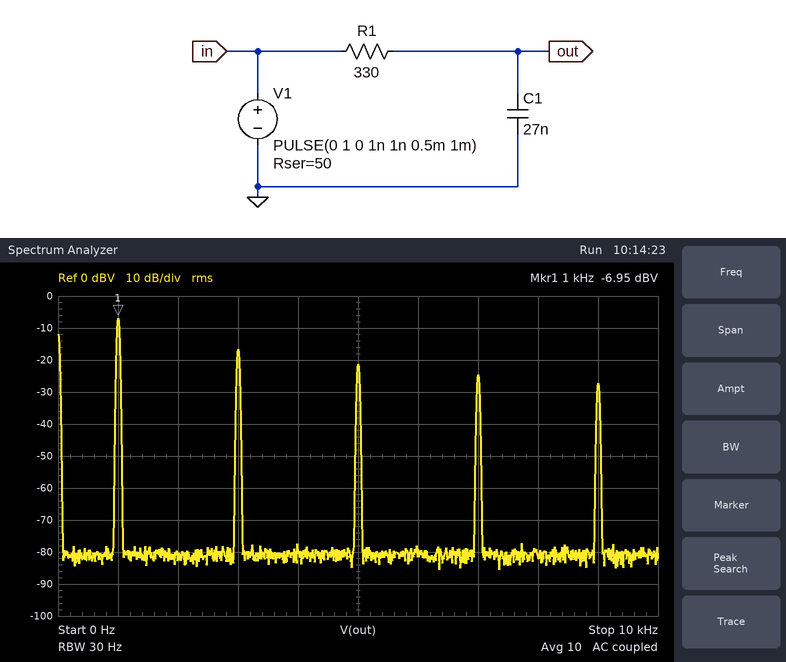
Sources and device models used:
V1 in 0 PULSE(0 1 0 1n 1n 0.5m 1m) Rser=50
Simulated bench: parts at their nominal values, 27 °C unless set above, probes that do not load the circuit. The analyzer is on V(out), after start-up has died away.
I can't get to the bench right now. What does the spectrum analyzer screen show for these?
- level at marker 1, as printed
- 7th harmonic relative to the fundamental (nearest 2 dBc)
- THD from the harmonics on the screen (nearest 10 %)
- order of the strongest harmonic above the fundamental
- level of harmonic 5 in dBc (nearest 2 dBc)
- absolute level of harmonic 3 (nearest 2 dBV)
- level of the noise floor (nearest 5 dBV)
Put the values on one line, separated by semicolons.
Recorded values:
-6.95 dBV; -18 dBc; 40 %; 3; -14 dBc; -16 dBV; -80 dBV
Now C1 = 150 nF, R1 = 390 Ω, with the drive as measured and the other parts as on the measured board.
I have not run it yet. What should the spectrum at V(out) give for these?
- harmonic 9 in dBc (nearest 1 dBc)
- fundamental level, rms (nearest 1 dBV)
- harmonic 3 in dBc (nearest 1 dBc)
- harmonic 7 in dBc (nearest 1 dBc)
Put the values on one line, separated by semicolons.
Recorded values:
-30 dBc; -8 dBV; -13 dBc; -26 dBc
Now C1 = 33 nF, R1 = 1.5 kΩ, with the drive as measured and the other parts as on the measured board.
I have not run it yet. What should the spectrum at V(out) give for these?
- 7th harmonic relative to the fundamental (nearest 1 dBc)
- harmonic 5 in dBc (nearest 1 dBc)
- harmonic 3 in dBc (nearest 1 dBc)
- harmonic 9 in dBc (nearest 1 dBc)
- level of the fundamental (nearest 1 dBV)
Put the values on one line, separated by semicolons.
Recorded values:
-24 dBc; -19 dBc; -12 dBc; -28 dBc; -7 dBV
